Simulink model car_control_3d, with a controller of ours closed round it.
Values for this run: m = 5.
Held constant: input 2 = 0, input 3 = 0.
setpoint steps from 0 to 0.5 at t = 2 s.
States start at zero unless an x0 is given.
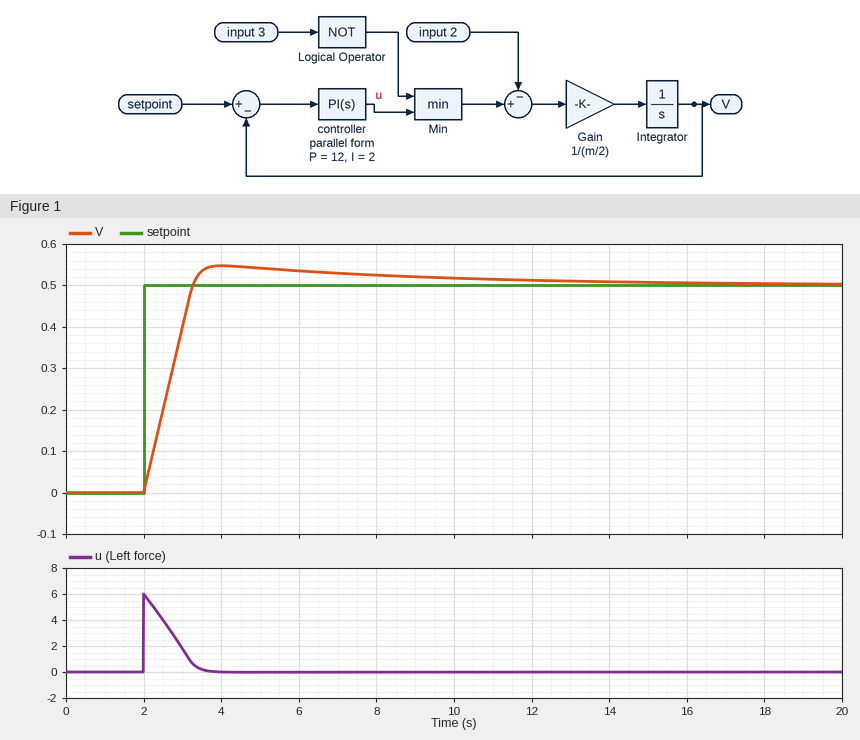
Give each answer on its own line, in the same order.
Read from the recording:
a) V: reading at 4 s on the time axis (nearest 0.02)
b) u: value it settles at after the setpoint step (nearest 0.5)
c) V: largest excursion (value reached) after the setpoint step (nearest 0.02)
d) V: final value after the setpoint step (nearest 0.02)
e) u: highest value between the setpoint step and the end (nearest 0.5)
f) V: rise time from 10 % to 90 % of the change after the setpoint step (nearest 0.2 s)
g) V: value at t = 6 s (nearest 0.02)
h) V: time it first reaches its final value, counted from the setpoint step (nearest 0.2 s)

0.54
0.0
0.54
0.50
6.0
1.0 s
0.54
1.2 s
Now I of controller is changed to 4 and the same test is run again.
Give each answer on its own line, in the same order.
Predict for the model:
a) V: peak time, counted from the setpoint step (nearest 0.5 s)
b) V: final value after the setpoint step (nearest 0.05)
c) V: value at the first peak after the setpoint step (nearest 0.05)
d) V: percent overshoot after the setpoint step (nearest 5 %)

2.0 s
0.50
0.60
20 %
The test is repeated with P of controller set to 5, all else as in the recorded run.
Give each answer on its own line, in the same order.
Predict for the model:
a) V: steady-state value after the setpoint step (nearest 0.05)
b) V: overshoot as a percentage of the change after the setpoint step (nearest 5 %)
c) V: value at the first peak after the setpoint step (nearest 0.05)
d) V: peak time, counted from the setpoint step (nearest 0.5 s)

0.50
20 %
0.60
2.5 s
